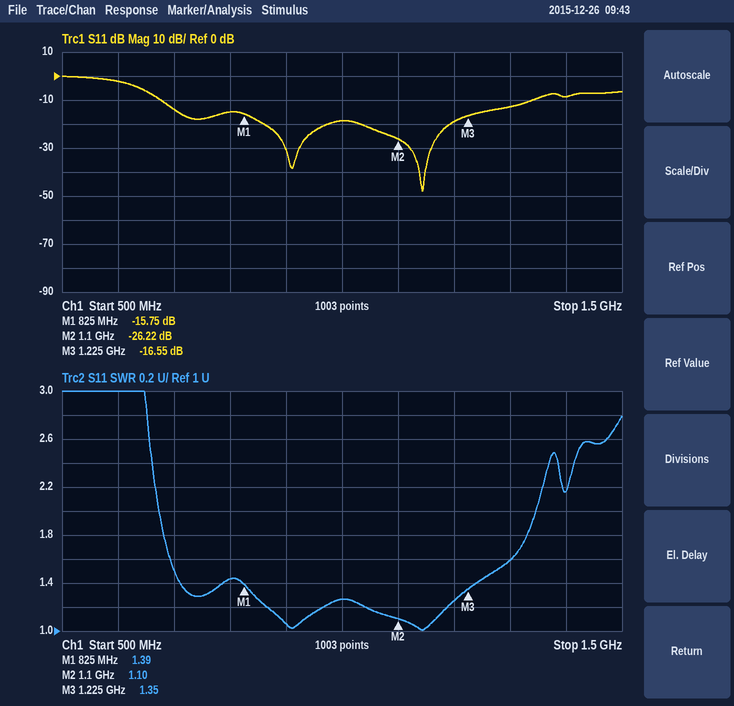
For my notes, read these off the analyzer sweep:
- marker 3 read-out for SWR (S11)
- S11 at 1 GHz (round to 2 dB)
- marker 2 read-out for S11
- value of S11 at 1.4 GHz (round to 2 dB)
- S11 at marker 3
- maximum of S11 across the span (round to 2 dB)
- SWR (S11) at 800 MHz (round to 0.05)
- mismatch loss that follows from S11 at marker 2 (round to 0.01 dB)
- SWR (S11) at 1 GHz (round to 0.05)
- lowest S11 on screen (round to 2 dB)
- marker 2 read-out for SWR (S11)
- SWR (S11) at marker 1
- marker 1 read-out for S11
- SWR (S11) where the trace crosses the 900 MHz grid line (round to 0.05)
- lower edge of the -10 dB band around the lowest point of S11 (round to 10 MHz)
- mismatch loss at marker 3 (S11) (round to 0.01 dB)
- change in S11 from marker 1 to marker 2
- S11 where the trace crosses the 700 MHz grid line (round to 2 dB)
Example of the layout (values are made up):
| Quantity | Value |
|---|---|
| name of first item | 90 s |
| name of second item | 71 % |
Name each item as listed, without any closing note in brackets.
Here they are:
| Quantity | Value |
|---|---|
| marker 3 read-out for SWR | 1.35 |
| S11 at 1 GHz | -18 dB |
| marker 2 read-out for S11 | -26.22 dB |
| value of S11 at 1.4 GHz | -8 dB |
| S11 at marker 3 | -16.55 dB |
| maximum of S11 across the span | 0 dB |
| SWR (S11) at 800 MHz | 1.45 |
| mismatch loss that follows from S11 at marker 2 | 0.01 dB |
| SWR (S11) at 1 GHz | 1.25 |
| lowest S11 on screen | -48 dB |
| marker 2 read-out for SWR | 1.10 |
| SWR (S11) at marker 1 | 1.39 |
| marker 1 read-out for S11 | -15.75 dB |
| SWR (S11) where the trace crosses the 900 MHz grid line | 1.05 |
| lower edge of the -10 dB band around the lowest point of S11 | 680 MHz |
| mismatch loss at marker 3 (S11) | 0.10 dB |
| change in S11 from marker 1 to marker 2 | -10.47 dB |
| S11 where the trace crosses the 700 MHz grid line | -14 dB |
